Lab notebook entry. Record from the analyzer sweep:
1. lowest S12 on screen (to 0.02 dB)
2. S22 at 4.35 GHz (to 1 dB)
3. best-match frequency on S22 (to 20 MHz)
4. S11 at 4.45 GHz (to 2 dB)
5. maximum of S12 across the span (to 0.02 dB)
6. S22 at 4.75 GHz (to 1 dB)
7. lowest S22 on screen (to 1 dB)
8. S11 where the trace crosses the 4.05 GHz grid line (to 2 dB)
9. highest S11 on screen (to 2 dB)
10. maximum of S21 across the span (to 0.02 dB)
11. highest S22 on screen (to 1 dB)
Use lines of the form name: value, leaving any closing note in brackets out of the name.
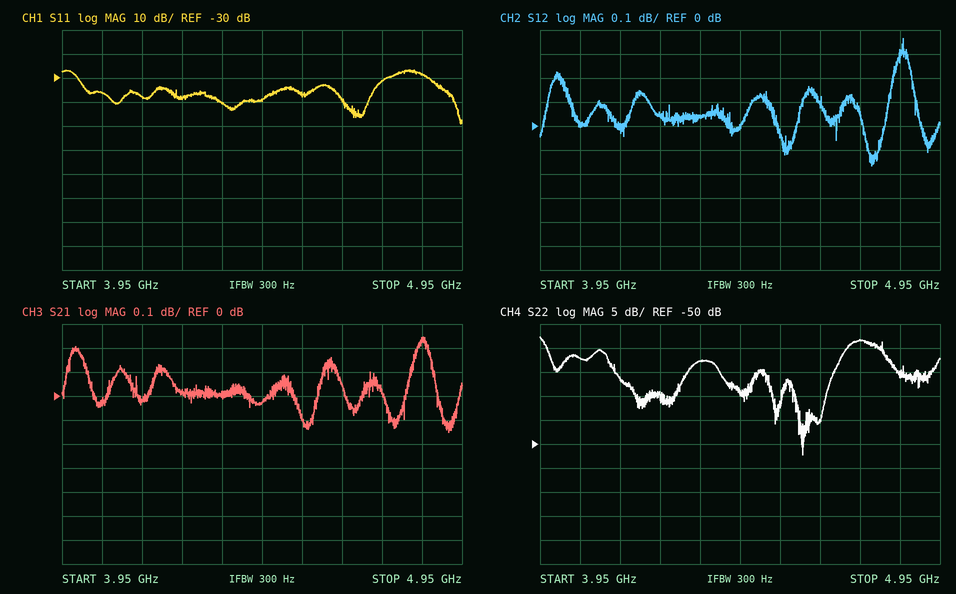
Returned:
lowest S12 on screen: -0.16 dB
S22 at 4.35 GHz: -33 dB
best-match frequency on S22: 4.60 GHz
S11 at 4.45 GHz: -40 dB
maximum of S12 across the span: 0.36 dB
S22 at 4.75 GHz: -28 dB
lowest S22 on screen: -52 dB
S11 where the trace crosses the 4.05 GHz grid line: -36 dB
highest S11 on screen: -26 dB
maximum of S21 across the span: 0.24 dB
highest S22 on screen: -28 dB
